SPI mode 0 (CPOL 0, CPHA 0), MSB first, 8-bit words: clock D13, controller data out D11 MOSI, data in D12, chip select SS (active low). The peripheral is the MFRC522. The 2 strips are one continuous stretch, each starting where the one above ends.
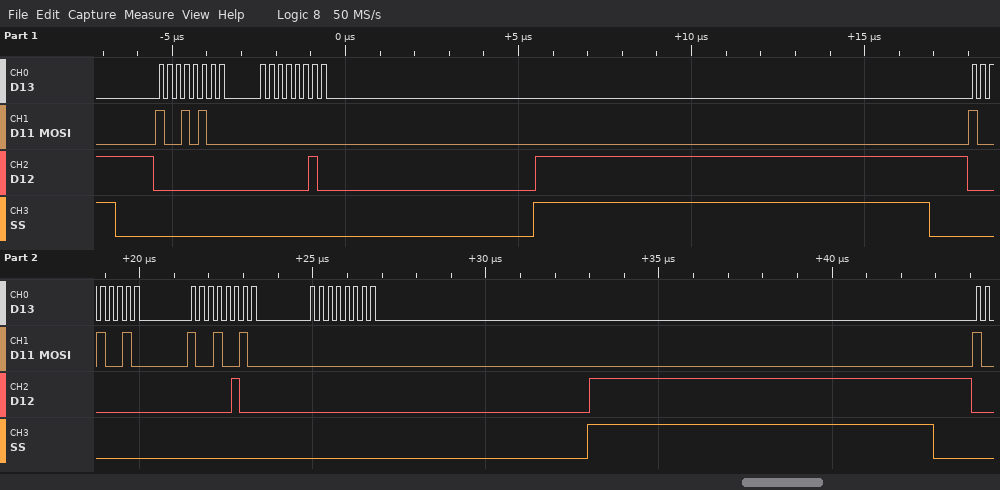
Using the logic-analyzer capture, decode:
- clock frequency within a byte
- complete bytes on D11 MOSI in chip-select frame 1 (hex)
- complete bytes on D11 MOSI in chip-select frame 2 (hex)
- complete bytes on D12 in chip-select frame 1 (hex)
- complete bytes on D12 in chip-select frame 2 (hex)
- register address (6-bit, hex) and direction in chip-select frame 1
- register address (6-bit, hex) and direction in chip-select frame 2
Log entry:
4 MHz
0x94 0x00
0x92 0x92 0x00
0x00 0x02
0x00 0x04 0x00
0x0A read
0x09 read
